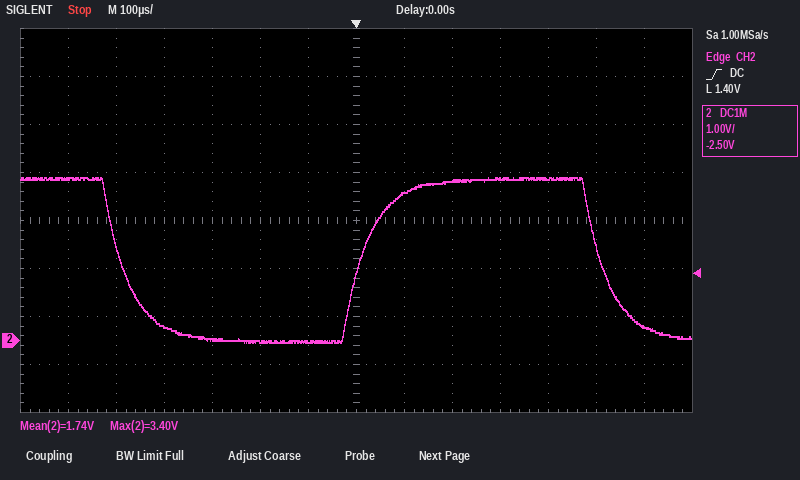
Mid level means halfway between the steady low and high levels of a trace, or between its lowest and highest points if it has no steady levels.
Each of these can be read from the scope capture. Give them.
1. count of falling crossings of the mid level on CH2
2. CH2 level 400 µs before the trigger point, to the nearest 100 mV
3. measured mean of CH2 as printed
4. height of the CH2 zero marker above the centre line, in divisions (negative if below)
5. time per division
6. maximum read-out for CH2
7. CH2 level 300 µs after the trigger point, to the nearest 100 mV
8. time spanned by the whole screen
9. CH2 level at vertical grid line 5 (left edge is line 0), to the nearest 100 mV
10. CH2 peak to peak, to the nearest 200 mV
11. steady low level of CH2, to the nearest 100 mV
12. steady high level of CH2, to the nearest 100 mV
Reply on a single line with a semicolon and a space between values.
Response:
2; 300 mV; 1.74 V; -2.5 div; 100 µs; 3.40 V; 3.4 V; 1.4 ms; 0.0 V; 3.4 V; 0.0 V; 3.4 V
